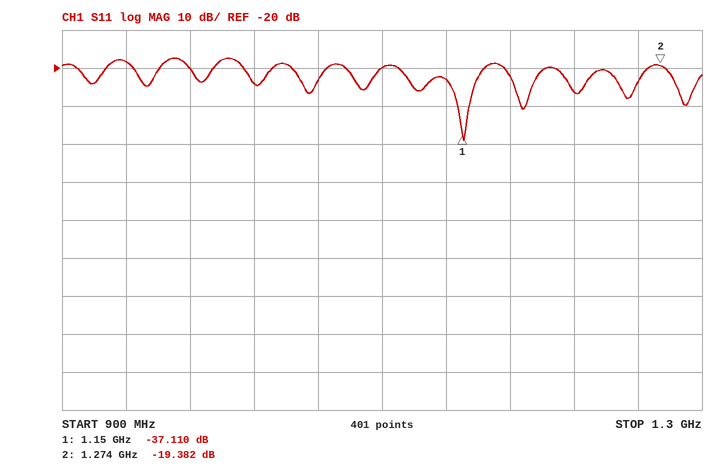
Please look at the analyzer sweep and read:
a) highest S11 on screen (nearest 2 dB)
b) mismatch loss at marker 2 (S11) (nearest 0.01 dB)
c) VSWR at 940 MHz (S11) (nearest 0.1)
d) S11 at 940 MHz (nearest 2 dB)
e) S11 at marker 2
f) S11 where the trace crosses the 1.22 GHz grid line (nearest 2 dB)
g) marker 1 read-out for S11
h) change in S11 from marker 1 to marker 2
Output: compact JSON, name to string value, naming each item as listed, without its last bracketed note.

{"highest S11 on screen": "-18 dB", "mismatch loss at marker 2 (S11)": "0.05 dB", "VSWR at 940 MHz (S11)": "1.3", "S11 at 940 MHz": "-18 dB", "S11 at marker 2": "-19.382 dB", "S11 where the trace crosses the 1.22 GHz grid line": "-26 dB", "marker 1 read-out for S11": "-37.110 dB", "change in S11 from marker 1 to marker 2": "17.728 dB"}
